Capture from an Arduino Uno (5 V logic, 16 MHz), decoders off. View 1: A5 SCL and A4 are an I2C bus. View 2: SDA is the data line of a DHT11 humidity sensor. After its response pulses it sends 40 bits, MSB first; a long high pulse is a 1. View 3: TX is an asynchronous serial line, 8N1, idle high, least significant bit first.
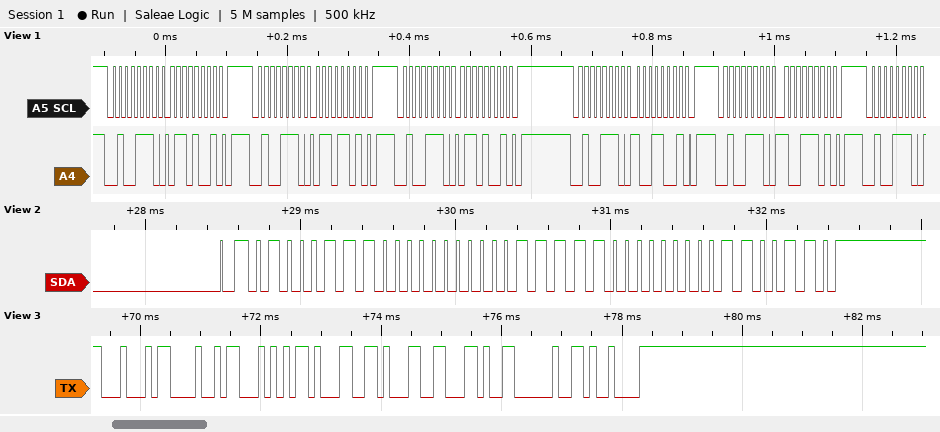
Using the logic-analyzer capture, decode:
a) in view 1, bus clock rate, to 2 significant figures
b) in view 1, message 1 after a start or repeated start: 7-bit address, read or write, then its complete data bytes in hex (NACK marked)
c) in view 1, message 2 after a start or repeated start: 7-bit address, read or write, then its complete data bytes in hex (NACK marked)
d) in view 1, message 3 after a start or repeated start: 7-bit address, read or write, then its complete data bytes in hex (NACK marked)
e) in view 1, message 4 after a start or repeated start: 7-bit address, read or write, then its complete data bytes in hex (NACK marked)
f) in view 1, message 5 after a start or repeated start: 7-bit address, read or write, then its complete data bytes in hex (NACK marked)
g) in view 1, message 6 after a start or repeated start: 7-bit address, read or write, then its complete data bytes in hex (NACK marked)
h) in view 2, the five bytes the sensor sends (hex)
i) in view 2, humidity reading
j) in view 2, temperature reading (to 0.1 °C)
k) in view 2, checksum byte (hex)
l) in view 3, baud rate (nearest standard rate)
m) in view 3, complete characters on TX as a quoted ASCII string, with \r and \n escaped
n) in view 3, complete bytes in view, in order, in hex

100 kHz
0x27 write: 69
0x27 write: 6D
0x27 write: 69
0x27 write: 99
0x27 write: 9D
0x27 write
47 00 1F 00 66
71 %
31.0 °C
0x66
9600 baud
"DHT11, \t"
44 48 54 31 31 2C 20 09
